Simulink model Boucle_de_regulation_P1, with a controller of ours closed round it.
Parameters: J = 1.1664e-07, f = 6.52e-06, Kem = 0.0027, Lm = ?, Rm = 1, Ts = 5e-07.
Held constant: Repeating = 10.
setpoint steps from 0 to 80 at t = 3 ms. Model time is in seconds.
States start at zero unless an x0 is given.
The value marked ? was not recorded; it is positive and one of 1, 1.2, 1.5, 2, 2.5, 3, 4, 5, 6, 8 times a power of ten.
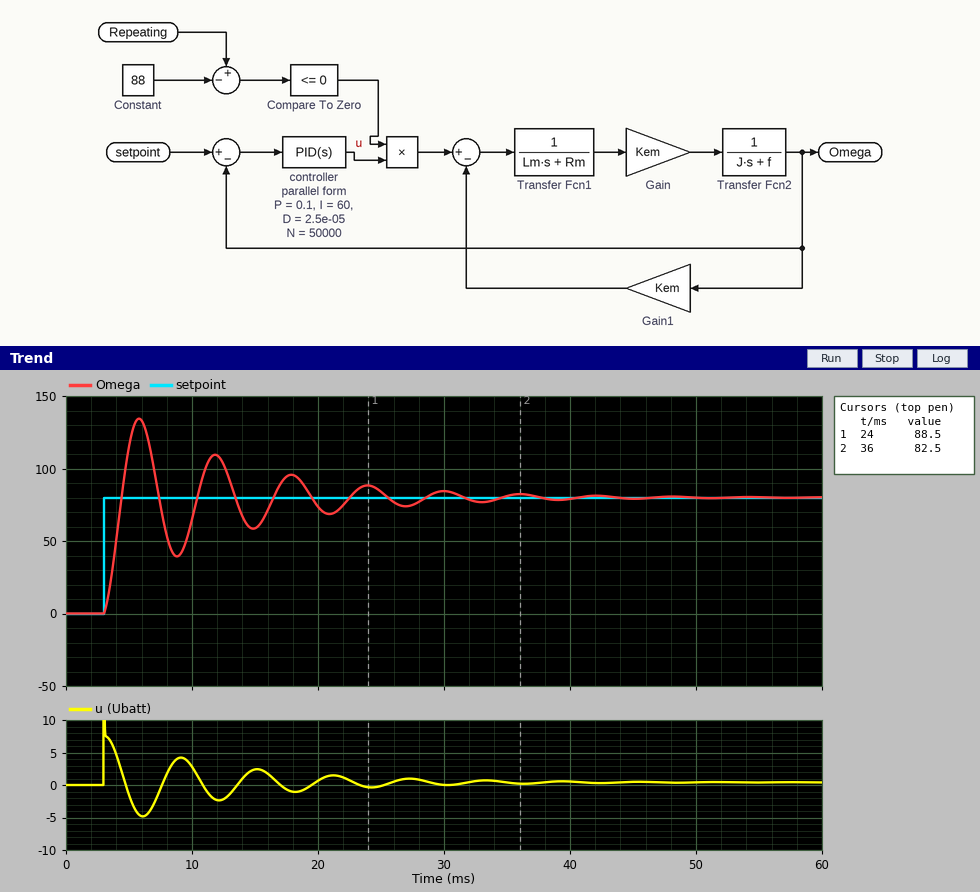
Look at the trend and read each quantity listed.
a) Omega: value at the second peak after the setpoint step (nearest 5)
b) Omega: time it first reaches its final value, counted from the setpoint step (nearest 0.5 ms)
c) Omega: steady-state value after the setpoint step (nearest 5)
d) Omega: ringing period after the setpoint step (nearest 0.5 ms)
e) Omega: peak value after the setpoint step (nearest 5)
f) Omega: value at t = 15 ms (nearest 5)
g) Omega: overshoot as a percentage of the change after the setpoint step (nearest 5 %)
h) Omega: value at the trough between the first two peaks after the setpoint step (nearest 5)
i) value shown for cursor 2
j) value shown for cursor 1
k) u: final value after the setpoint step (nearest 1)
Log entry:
110
1.5 ms
80
6.0 ms
135
60
70 %
40
82.5
88.5
0
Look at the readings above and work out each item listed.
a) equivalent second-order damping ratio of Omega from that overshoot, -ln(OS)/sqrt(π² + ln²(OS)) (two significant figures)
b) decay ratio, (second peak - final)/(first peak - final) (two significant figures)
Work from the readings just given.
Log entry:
0.11
0.55
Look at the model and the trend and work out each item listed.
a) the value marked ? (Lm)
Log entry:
0.002
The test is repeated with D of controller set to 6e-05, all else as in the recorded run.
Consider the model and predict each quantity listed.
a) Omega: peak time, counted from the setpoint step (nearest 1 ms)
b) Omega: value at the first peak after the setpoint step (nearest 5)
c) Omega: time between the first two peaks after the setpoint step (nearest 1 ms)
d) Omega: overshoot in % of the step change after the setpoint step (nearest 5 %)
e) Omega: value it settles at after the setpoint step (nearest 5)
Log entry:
3 ms
115
7 ms
45 %
80
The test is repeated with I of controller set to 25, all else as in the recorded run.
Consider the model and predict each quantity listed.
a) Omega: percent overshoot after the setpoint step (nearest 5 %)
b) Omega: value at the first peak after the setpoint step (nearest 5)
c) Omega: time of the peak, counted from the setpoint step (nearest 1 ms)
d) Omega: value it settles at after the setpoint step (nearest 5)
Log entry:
45 %
115
3 ms
80
